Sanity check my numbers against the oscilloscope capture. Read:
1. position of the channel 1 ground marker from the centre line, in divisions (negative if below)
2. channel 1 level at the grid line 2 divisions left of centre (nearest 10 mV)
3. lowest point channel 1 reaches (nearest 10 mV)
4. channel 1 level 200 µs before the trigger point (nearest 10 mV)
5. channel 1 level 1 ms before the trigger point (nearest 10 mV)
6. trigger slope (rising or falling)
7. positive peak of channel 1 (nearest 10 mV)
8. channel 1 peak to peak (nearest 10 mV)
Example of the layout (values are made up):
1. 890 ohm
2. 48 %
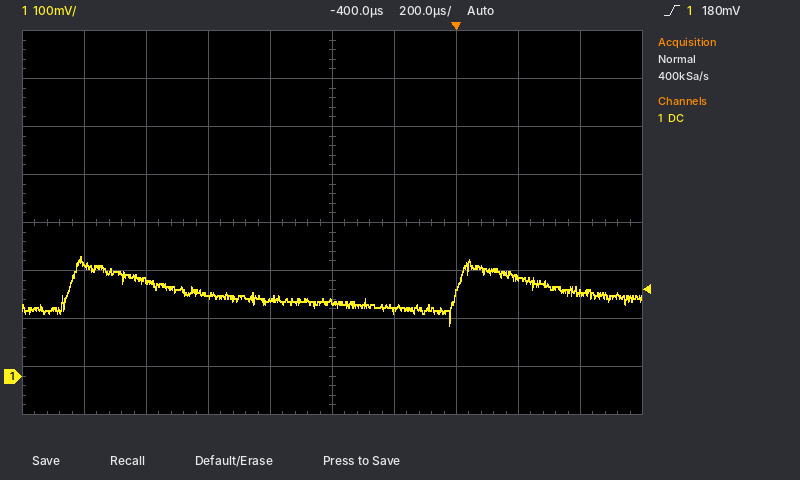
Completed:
1. -3.2 div
2. 170 mV
3. 110 mV
4. 140 mV
5. 200 mV
6. rising
7. 250 mV
8. 140 mV
